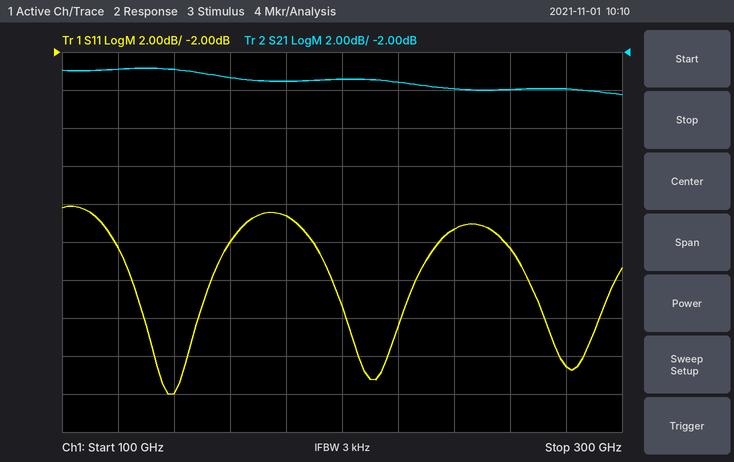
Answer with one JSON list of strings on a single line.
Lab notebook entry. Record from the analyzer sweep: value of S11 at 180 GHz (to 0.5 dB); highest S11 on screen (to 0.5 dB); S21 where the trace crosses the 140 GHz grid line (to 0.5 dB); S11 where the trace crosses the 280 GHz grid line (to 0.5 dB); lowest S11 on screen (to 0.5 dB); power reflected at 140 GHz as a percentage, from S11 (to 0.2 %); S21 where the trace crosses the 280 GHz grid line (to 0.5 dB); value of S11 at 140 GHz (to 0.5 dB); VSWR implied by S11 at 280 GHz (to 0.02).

["-10.5 dB", "-10.0 dB", "-3.0 dB", "-18.5 dB", "-20.0 dB", "1.0 %", "-4.0 dB", "-20.0 dB", "1.26"]
